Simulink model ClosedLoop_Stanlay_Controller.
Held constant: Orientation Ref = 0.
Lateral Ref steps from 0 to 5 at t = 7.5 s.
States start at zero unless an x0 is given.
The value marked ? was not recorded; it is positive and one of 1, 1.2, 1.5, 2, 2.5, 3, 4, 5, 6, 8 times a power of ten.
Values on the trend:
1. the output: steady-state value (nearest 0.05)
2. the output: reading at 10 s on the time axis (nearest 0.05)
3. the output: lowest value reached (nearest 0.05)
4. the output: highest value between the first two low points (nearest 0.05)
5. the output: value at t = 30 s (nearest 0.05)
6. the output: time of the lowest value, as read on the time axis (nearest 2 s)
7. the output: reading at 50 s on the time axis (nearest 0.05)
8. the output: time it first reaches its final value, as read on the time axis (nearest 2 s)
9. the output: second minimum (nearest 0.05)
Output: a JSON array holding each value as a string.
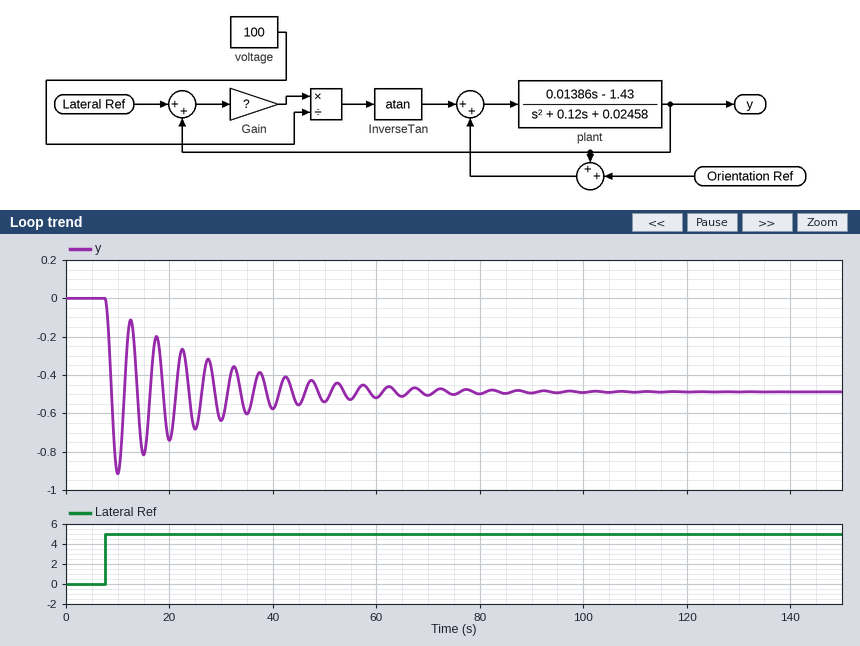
["-0.50", "-0.90", "-0.90", "-0.10", "-0.65", "10 s", "-0.55", "8 s", "-0.80"]
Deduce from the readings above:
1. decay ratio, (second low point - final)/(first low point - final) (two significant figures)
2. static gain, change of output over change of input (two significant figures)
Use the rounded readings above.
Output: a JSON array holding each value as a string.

["0.75", "-0.10"]
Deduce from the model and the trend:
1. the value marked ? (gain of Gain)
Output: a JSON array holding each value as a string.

["12"]
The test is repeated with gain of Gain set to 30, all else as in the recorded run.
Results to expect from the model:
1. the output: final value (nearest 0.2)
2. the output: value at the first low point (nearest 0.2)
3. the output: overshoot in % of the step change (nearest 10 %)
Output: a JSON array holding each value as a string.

["-0.8", "-1.6", "90 %"]
